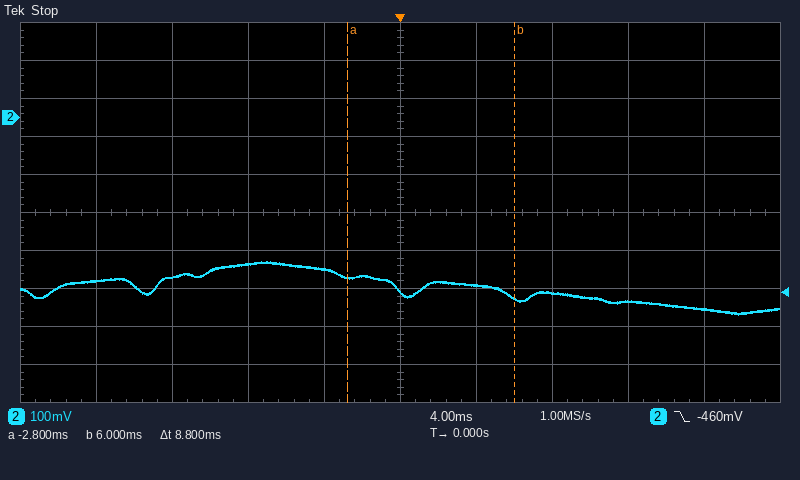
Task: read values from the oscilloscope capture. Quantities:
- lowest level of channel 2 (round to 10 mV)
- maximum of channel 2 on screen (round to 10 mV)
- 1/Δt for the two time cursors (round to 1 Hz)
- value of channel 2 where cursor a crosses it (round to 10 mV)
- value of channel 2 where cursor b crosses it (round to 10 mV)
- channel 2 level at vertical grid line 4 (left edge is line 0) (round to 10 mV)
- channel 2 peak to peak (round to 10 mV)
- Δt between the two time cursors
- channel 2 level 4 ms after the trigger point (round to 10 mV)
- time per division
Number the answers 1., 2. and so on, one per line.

1. -520 mV
2. -380 mV
3. 114 Hz
4. -420 mV
5. -480 mV
6. -400 mV
7. 140 mV
8. 8.8 ms
9. -440 mV
10. 4 ms
